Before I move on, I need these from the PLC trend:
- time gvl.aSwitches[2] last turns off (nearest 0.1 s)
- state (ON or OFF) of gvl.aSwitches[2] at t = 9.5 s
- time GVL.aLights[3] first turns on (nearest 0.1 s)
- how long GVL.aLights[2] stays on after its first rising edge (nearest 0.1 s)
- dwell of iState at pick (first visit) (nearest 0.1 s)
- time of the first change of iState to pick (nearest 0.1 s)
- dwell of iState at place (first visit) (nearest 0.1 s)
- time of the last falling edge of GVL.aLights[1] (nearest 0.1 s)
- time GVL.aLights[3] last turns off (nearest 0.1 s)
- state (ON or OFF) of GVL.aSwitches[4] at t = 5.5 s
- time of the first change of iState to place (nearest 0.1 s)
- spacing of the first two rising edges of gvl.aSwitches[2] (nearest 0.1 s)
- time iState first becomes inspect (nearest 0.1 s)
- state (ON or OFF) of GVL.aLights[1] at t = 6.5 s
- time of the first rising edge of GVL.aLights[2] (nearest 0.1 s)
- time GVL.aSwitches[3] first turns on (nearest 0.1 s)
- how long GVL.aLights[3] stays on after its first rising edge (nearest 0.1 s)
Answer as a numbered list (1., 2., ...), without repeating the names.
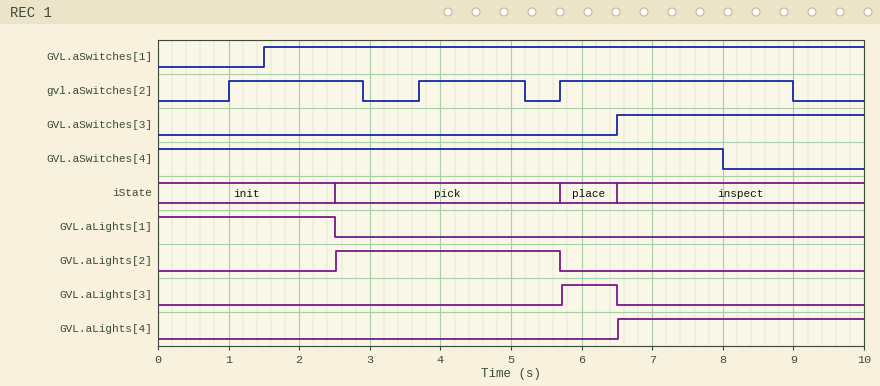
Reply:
1. 9.0 s
2. OFF
3. 5.7 s
4. 3.2 s
5. 3.2 s
6. 2.5 s
7. 0.8 s
8. 2.5 s
9. 6.5 s
10. ON
11. 5.7 s
12. 2.7 s
13. 6.5 s
14. OFF
15. 2.5 s
16. 6.5 s
17. 0.8 s
